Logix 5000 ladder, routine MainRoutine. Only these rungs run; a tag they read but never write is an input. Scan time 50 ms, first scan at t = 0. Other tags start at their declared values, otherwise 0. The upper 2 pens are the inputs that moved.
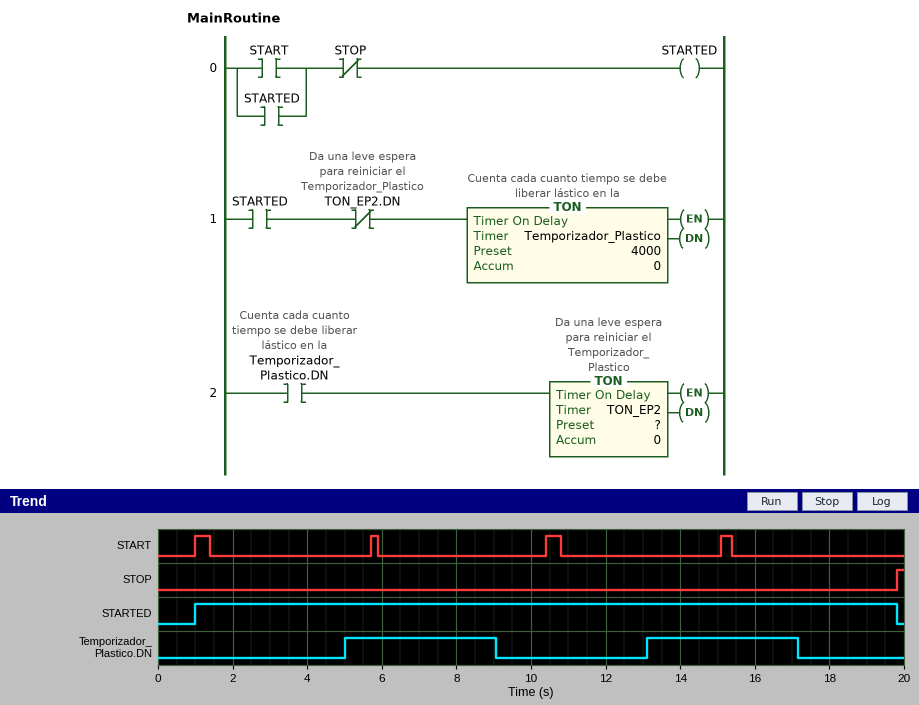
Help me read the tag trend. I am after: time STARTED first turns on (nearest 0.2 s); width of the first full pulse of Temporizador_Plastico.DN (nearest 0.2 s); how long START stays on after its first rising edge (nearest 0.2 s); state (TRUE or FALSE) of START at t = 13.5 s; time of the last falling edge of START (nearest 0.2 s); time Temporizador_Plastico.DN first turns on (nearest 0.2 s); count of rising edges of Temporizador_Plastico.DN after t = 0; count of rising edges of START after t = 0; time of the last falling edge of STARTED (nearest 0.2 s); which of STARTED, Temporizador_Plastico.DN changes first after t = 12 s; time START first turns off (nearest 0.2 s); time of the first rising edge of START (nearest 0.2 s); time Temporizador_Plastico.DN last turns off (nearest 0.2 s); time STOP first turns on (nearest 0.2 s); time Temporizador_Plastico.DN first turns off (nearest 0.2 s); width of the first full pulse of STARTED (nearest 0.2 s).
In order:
1.0 s
4.0 s
0.4 s
FALSE
15.4 s
5.0 s
2
4
19.8 s
Temporizador_Plastico.DN
1.4 s
1.0 s
17.2 s
19.8 s
9.0 s
18.8 s
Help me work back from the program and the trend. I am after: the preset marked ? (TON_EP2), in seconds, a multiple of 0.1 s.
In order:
4.0 s
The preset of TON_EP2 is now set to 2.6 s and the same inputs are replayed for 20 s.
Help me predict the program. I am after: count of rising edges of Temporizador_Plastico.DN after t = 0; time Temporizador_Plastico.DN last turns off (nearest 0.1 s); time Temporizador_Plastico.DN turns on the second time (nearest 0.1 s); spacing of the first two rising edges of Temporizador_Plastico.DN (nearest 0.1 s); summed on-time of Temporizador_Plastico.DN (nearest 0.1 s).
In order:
3
19.8 s
11.7 s
6.7 s
6.7 s
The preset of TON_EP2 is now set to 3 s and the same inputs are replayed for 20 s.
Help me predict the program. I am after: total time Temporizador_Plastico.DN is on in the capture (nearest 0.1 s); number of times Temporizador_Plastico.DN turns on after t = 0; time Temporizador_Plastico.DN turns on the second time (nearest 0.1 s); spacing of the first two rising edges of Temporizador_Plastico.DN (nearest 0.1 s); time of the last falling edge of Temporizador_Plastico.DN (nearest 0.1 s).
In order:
6.7 s
3
12.1 s
7.1 s
19.8 s
